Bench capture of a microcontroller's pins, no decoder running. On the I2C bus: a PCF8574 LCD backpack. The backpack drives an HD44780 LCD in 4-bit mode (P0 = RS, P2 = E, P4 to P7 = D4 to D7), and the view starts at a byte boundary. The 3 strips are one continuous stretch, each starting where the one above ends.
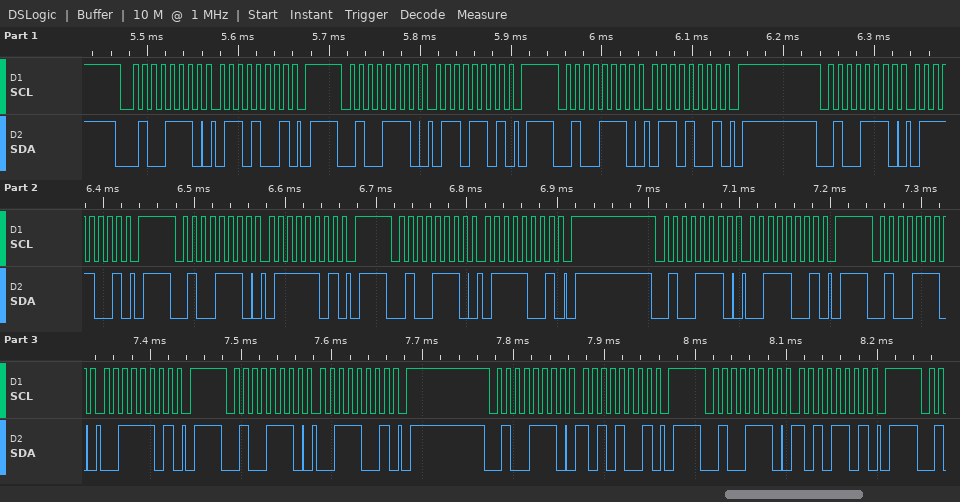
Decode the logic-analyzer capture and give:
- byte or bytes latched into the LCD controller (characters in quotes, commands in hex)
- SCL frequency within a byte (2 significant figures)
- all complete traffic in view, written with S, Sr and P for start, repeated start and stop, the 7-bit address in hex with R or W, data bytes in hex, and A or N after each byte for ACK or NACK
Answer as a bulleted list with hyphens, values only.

- 'g'
- 100 kHz
- S 27W A 69 A P S 27W A 6D A P S 27W A 69 A P S 27W A 79 A P S 27W A 7D A P S 27W A 79 A P S 27W A 39 A P S 27W A 3D A P S 27W A 39 A P S 27W A A9 A P S 27W A AD A P
